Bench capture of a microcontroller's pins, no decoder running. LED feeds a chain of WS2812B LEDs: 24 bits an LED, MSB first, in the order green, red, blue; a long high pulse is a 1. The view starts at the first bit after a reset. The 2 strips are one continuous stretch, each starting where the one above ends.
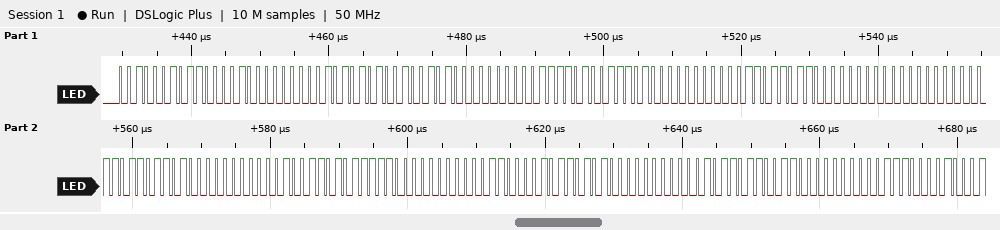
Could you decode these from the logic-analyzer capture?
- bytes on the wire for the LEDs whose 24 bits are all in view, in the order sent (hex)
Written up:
22 C2 00 AA 4A 00 7A 74 00 6D 80 00 06 DA 00 26 BE 00 30 B5 00 16 CC 00
